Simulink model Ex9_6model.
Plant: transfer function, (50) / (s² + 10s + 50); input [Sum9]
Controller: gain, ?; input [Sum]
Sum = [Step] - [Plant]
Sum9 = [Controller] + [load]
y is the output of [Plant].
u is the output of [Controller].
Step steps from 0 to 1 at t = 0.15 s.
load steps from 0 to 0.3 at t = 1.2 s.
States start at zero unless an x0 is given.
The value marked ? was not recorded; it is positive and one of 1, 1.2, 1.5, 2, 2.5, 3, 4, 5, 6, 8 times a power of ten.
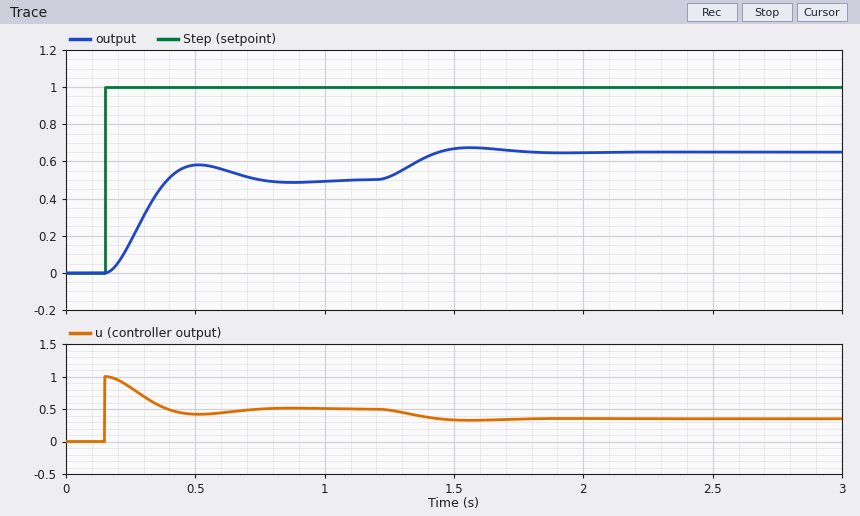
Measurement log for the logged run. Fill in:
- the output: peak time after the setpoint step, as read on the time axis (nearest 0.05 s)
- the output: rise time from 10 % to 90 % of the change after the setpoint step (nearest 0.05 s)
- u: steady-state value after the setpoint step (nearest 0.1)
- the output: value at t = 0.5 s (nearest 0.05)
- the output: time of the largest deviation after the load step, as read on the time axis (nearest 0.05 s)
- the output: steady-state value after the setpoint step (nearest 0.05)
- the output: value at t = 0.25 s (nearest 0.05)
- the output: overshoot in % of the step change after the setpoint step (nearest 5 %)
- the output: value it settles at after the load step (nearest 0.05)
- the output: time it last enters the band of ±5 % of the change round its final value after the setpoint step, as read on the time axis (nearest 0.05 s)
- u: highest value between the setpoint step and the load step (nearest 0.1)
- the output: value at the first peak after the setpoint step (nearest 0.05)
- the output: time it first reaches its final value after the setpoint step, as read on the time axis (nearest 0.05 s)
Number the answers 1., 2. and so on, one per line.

1. 0.50 s
2. 0.15 s
3. 0.5
4. 0.60
5. 1.55 s
6. 0.50
7. 0.15
8. 15 %
9. 0.65
10. 0.70 s
11. 1.0
12. 0.60
13. 0.40 s
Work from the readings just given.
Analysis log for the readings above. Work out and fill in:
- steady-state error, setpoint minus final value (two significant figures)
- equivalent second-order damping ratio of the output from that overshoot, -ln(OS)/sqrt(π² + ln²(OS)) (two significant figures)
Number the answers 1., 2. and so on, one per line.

1. 0.50
2. 0.52
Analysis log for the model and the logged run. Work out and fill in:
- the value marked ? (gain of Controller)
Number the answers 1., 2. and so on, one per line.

1. 1
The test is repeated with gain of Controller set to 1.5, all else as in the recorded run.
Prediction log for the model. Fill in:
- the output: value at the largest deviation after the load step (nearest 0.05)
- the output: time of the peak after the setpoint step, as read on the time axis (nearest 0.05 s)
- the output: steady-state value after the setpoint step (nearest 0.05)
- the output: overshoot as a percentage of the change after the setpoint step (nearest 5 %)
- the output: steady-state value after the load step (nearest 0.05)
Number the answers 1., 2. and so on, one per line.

1. 0.75
2. 0.45 s
3. 0.60
4. 20 %
5. 0.70
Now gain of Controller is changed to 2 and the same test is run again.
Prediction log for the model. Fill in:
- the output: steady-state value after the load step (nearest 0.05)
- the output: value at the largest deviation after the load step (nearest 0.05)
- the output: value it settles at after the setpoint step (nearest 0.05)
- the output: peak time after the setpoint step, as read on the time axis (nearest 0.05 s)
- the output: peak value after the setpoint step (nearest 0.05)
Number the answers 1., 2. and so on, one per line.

1. 0.75
2. 0.80
3. 0.65
4. 0.45 s
5. 0.85
